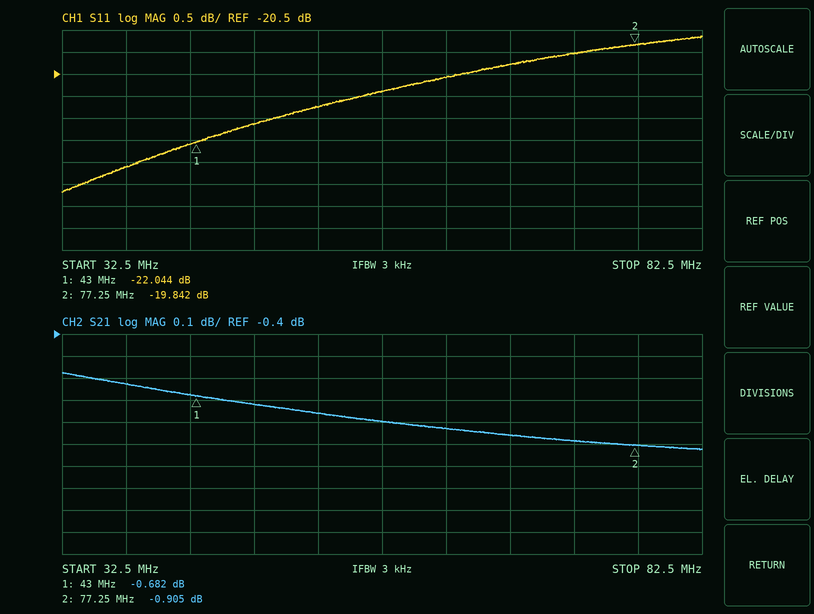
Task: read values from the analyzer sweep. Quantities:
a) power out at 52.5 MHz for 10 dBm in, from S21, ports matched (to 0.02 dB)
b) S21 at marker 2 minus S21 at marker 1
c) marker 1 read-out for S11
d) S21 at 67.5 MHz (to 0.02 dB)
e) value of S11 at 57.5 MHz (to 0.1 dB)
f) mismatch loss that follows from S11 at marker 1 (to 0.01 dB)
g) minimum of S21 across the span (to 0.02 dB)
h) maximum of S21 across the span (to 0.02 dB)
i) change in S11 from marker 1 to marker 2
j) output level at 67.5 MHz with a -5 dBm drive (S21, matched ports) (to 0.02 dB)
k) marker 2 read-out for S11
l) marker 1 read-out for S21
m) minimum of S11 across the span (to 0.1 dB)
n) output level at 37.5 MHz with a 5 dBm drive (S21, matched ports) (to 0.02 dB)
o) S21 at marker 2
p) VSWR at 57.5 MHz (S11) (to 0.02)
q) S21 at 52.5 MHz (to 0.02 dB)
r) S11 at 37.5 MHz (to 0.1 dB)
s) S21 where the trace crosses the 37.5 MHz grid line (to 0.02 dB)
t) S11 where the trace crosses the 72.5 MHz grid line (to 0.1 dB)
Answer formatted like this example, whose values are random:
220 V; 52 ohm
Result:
9.24 dBm; -0.223 dB; -22.044 dB; -0.86 dB; -20.9 dB; 0.03 dB; -0.92 dB; -0.58 dB; 2.202 dB; -5.86 dBm; -19.842 dB; -0.682 dB; -23.2 dB; 4.38 dBm; -0.905 dB; 1.20; -0.76 dB; -22.6 dB; -0.62 dB; -20.0 dB
